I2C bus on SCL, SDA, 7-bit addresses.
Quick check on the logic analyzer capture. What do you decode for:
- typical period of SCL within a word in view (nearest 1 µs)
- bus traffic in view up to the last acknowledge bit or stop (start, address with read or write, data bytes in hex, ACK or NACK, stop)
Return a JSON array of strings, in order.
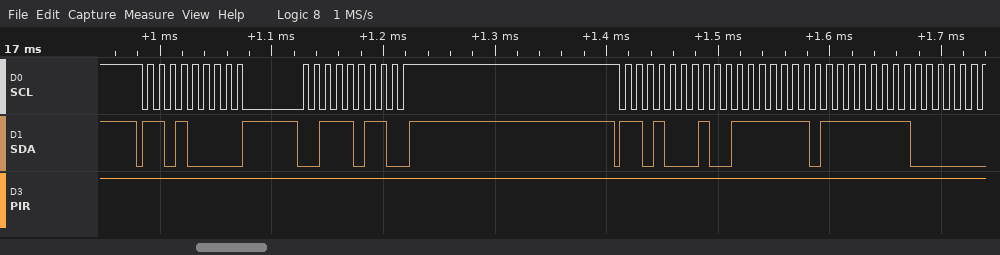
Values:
["10 µs", "start, address 68 write ACK, 3B ACK, stop, start, address 68 read ACK, 7F ACK, FF ACK"]
